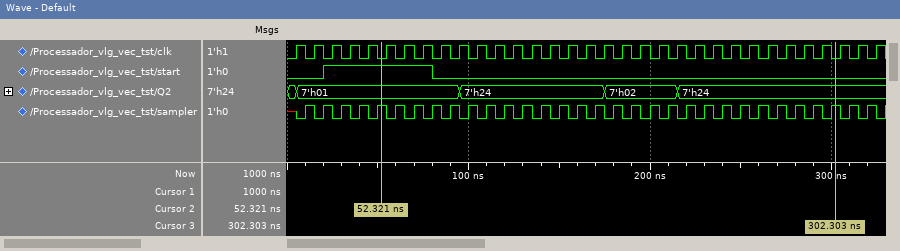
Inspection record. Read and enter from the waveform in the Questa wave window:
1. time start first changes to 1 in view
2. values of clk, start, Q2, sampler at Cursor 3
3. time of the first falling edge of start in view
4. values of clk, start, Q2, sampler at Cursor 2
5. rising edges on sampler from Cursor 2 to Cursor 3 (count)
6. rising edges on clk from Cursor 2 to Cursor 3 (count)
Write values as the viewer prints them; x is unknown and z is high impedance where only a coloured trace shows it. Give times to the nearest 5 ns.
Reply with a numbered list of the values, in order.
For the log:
1. 20 ns
2. clk=0, start=0, Q2=7'h24, sampler=1
3. 80 ns
4. clk=0, start=1, Q2=7'h01, sampler=1
5. 25
6. 25
